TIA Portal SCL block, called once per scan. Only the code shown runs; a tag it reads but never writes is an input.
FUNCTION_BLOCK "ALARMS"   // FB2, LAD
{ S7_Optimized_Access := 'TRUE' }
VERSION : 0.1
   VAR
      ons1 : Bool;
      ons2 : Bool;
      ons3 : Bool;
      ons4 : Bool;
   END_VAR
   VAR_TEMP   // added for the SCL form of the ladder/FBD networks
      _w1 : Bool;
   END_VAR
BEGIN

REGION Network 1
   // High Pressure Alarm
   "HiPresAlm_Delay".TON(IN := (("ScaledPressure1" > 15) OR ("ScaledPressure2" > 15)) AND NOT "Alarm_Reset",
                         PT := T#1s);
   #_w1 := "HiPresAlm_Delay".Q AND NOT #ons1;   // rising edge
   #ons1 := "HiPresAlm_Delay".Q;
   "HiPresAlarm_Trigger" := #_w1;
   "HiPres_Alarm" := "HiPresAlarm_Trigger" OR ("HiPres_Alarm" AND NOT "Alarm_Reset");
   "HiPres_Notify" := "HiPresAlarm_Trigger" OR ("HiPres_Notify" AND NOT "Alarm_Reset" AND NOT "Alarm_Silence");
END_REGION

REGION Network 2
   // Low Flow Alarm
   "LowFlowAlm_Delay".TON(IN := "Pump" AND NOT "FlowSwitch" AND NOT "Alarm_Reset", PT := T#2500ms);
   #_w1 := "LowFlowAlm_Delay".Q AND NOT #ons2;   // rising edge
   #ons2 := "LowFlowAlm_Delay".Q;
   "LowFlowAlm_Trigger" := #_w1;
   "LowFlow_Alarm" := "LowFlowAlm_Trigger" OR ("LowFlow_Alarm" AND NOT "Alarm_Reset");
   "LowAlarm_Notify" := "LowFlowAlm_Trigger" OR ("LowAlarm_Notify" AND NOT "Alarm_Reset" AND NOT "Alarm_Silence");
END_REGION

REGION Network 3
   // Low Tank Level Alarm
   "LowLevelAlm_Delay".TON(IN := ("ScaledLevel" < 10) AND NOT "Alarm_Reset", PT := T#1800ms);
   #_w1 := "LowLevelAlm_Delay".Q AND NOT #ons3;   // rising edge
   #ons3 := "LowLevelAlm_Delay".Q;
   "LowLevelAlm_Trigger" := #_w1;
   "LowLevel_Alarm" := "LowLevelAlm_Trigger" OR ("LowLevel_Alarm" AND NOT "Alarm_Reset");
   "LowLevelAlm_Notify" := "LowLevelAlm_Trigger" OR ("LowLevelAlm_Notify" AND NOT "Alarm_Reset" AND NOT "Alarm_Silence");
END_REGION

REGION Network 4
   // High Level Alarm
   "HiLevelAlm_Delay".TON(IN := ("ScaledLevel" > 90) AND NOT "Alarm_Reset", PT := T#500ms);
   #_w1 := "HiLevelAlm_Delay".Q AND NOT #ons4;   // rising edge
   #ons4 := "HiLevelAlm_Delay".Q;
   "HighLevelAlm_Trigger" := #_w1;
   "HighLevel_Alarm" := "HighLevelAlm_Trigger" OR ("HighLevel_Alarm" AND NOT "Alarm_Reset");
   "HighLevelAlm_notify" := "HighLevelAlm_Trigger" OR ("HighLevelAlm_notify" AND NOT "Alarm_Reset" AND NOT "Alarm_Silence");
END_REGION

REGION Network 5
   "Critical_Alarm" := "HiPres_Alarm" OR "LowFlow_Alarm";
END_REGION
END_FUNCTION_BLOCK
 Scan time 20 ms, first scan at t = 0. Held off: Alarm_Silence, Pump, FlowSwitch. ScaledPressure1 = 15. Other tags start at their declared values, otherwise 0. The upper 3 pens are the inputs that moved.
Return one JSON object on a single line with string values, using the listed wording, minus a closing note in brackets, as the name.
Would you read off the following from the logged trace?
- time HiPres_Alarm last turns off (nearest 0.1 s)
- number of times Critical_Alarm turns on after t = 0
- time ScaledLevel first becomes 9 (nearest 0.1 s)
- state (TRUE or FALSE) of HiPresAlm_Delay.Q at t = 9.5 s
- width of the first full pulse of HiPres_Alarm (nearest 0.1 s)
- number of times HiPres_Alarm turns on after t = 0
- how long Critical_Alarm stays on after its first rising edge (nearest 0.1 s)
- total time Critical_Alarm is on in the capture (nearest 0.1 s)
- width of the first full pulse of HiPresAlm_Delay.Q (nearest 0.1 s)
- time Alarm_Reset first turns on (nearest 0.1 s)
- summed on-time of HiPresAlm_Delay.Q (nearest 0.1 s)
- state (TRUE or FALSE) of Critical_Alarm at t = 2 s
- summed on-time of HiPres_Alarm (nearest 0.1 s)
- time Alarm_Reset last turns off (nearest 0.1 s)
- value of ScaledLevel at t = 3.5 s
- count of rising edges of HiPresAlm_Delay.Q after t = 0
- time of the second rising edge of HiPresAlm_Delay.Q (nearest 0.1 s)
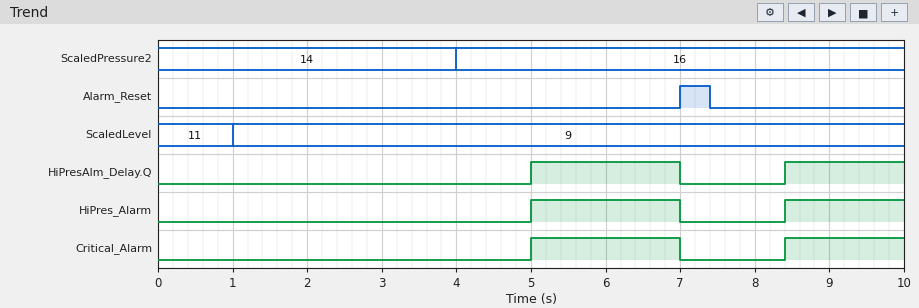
{"time HiPres_Alarm last turns off": "7.0 s", "number of times Critical_Alarm turns on after t = 0": "2", "time ScaledLevel first becomes 9": "1.0 s", "state (TRUE or FALSE) of HiPresAlm_Delay.Q at t = 9.5 s": "TRUE", "width of the first full pulse of HiPres_Alarm": "2.0 s", "number of times HiPres_Alarm turns on after t = 0": "2", "how long Critical_Alarm stays on after its first rising edge": "2.0 s", "total time Critical_Alarm is on in the capture": "3.6 s", "width of the first full pulse of HiPresAlm_Delay.Q": "2.0 s", "time Alarm_Reset first turns on": "7.0 s", "summed on-time of HiPresAlm_Delay.Q": "3.6 s", "state (TRUE or FALSE) of Critical_Alarm at t = 2 s": "FALSE", "summed on-time of HiPres_Alarm": "3.6 s", "time Alarm_Reset last turns off": "7.4 s", "value of ScaledLevel at t = 3.5 s": "9", "count of rising edges of HiPresAlm_Delay.Q after t = 0": "2", "time of the second rising edge of HiPresAlm_Delay.Q": "8.4 s"}
